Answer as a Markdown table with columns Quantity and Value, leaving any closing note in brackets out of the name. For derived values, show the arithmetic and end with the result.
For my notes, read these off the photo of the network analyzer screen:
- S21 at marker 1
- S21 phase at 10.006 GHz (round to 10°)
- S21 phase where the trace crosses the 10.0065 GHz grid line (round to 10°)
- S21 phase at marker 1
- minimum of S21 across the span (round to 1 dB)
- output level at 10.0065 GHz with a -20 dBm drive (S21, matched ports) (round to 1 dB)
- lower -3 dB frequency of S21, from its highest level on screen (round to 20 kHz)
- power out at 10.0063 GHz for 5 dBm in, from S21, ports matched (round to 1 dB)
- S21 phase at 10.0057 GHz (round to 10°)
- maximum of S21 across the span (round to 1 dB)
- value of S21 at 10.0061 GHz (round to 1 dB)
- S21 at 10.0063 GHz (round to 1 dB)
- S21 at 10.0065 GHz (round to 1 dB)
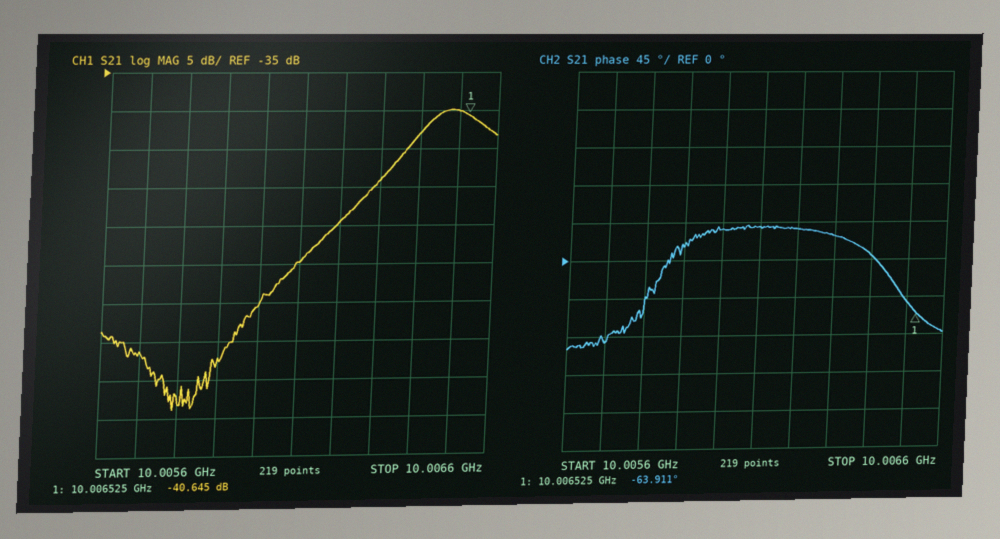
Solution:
| Quantity | Value |
|---|---|
| S21 at marker 1 | -40.645 dB |
| S21 phase at 10.006 GHz | 40° |
| S21 phase where the trace crosses the 10.0065 GHz grid line | -50° |
| S21 phase at marker 1 | -63.911° |
| minimum of S21 across the span | -79 dB |
| output level at 10.0065 GHz with a -20 dBm drive (S21, matched ports) | -20 dBm + (-40 dB) = -60 dBm |
| lower -3 dB frequency of S21, from its highest level on screen | 10.00640 GHz |
| power out at 10.0063 GHz for 5 dBm in, from S21, ports matched | 5 dBm + (-49 dB) = -44 dBm |
| S21 phase at 10.0057 GHz | -100° |
| maximum of S21 across the span | -40 dB |
| value of S21 at 10.0061 GHz | -60 dB |
| S21 at 10.0063 GHz | -49 dB |
| S21 at 10.0065 GHz | -40 dB |
